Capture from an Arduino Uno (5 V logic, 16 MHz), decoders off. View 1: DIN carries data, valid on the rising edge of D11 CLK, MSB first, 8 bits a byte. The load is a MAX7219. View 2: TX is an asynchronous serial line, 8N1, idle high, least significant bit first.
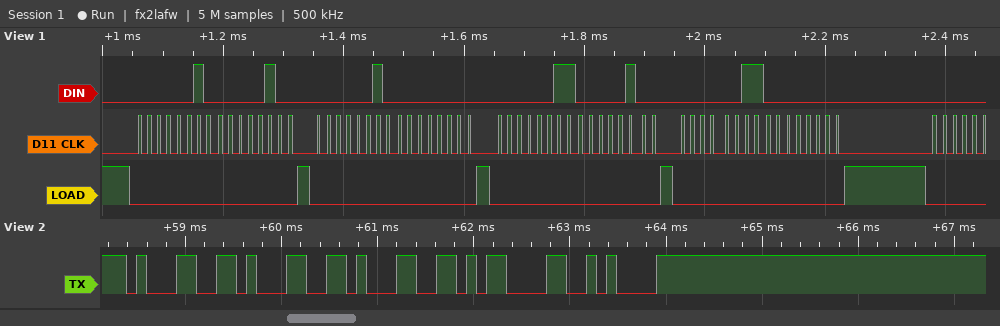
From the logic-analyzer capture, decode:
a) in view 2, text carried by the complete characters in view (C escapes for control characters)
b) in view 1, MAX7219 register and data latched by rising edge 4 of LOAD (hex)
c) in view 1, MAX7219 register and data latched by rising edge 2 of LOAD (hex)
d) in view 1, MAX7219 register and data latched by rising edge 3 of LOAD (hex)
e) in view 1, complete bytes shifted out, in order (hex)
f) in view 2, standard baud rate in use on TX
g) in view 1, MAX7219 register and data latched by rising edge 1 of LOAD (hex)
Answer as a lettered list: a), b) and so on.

a) "111\r\n"
b) register 0x3, data 0x00
c) register 0x2, data 0x00
d) register 0x3, data 0x04
e) 02 04 02 00 03 04 03 00
f) 9600 baud
g) register 0x2, data 0x04
